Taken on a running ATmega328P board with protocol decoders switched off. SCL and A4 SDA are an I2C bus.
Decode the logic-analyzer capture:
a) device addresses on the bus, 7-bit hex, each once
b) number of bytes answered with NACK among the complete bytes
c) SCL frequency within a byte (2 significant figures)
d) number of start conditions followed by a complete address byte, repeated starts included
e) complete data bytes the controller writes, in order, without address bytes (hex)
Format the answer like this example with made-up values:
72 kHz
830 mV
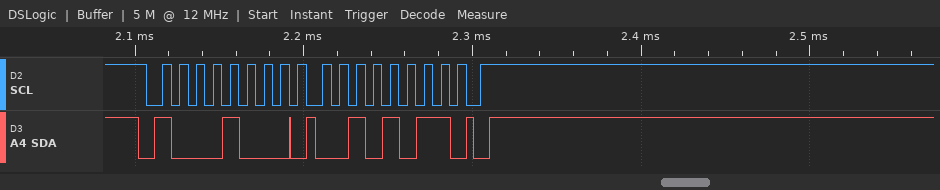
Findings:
0x44
0
100 kHz
1
2B
